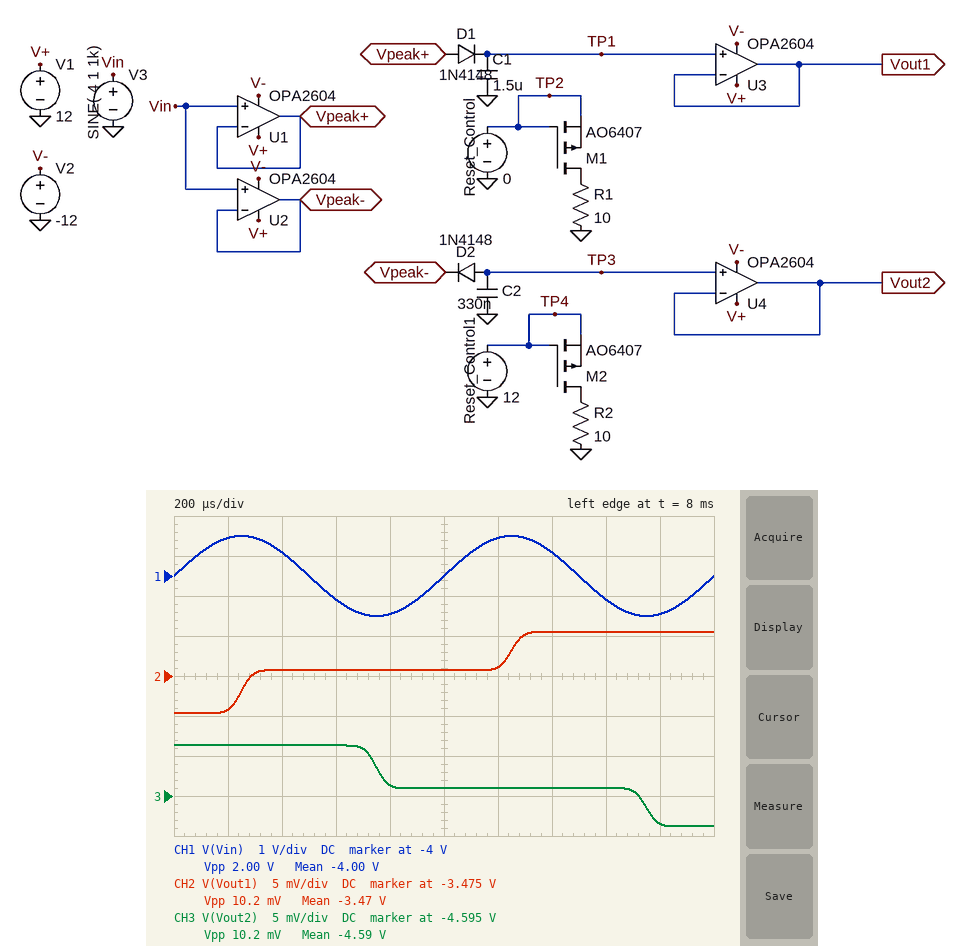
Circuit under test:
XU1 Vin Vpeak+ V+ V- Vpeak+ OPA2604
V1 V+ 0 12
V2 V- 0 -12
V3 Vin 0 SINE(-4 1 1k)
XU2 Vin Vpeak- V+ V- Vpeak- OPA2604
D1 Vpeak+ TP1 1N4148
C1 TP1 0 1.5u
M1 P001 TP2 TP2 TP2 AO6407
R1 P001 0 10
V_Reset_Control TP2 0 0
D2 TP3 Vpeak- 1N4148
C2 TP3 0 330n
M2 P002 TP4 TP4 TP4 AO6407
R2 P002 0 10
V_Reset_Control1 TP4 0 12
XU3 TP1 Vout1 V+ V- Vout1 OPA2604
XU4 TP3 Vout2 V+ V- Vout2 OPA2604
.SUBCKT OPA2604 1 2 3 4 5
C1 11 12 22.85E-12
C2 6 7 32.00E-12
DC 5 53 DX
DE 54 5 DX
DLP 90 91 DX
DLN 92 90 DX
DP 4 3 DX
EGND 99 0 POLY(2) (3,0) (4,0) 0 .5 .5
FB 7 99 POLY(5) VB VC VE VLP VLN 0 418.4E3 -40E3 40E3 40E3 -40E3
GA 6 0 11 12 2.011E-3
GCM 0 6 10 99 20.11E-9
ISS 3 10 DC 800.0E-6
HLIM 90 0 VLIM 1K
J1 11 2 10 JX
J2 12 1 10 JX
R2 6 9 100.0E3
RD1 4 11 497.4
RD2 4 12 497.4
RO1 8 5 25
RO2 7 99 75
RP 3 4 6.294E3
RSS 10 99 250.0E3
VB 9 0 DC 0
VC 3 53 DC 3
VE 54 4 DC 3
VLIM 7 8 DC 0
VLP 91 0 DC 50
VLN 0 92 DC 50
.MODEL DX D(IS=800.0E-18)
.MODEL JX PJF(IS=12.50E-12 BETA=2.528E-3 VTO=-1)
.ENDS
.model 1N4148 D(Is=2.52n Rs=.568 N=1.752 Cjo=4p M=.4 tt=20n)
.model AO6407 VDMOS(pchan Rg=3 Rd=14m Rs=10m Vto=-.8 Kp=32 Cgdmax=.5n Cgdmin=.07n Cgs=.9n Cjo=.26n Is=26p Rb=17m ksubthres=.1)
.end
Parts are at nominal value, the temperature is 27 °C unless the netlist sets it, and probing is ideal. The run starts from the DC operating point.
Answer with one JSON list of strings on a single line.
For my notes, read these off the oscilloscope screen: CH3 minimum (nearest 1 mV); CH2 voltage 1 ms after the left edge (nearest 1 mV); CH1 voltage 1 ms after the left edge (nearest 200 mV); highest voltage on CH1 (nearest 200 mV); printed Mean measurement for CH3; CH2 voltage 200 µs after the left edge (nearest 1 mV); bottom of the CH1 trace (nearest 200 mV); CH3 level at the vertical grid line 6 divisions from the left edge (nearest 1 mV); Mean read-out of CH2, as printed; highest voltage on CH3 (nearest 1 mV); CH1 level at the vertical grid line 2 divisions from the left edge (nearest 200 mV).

["-4.599 V", "-3.474 V", "-4.0 V", "-3.0 V", "-4.59 V", "-3.479 V", "-5.0 V", "-4.594 V", "-3.47 V", "-4.589 V", "-3.4 V"]
